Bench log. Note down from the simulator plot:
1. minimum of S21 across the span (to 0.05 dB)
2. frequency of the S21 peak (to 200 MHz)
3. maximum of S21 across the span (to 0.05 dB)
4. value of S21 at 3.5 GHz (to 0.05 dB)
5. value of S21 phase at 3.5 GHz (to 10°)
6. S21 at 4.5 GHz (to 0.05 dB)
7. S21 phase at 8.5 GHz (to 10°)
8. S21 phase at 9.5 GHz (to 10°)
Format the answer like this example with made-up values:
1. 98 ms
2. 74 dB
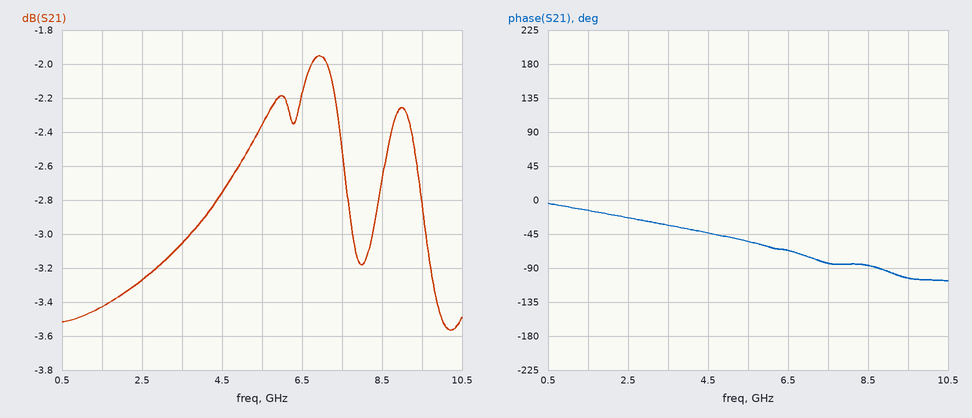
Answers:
1. -3.55 dB
2. 7.0 GHz
3. -1.95 dB
4. -3.05 dB
5. -30°
6. -2.75 dB
7. -90°
8. -100°
